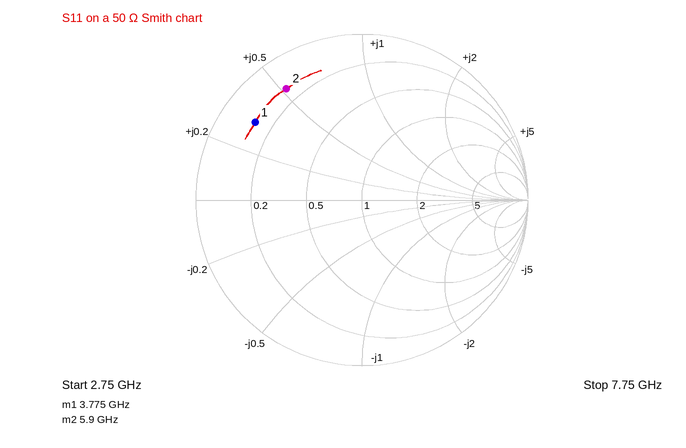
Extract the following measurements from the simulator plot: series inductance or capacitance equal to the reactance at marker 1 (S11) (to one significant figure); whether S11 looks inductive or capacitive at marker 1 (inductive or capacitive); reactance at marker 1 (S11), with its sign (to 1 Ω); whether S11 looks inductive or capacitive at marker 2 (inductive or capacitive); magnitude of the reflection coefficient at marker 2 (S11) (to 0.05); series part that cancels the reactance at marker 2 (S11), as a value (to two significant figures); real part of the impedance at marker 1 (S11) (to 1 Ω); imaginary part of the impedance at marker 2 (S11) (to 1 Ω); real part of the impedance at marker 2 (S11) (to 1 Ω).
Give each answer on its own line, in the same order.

700 pH
inductive
+16 Ω
inductive
0.80
1.0 pF
6 Ω
+26 Ω
7 Ω
